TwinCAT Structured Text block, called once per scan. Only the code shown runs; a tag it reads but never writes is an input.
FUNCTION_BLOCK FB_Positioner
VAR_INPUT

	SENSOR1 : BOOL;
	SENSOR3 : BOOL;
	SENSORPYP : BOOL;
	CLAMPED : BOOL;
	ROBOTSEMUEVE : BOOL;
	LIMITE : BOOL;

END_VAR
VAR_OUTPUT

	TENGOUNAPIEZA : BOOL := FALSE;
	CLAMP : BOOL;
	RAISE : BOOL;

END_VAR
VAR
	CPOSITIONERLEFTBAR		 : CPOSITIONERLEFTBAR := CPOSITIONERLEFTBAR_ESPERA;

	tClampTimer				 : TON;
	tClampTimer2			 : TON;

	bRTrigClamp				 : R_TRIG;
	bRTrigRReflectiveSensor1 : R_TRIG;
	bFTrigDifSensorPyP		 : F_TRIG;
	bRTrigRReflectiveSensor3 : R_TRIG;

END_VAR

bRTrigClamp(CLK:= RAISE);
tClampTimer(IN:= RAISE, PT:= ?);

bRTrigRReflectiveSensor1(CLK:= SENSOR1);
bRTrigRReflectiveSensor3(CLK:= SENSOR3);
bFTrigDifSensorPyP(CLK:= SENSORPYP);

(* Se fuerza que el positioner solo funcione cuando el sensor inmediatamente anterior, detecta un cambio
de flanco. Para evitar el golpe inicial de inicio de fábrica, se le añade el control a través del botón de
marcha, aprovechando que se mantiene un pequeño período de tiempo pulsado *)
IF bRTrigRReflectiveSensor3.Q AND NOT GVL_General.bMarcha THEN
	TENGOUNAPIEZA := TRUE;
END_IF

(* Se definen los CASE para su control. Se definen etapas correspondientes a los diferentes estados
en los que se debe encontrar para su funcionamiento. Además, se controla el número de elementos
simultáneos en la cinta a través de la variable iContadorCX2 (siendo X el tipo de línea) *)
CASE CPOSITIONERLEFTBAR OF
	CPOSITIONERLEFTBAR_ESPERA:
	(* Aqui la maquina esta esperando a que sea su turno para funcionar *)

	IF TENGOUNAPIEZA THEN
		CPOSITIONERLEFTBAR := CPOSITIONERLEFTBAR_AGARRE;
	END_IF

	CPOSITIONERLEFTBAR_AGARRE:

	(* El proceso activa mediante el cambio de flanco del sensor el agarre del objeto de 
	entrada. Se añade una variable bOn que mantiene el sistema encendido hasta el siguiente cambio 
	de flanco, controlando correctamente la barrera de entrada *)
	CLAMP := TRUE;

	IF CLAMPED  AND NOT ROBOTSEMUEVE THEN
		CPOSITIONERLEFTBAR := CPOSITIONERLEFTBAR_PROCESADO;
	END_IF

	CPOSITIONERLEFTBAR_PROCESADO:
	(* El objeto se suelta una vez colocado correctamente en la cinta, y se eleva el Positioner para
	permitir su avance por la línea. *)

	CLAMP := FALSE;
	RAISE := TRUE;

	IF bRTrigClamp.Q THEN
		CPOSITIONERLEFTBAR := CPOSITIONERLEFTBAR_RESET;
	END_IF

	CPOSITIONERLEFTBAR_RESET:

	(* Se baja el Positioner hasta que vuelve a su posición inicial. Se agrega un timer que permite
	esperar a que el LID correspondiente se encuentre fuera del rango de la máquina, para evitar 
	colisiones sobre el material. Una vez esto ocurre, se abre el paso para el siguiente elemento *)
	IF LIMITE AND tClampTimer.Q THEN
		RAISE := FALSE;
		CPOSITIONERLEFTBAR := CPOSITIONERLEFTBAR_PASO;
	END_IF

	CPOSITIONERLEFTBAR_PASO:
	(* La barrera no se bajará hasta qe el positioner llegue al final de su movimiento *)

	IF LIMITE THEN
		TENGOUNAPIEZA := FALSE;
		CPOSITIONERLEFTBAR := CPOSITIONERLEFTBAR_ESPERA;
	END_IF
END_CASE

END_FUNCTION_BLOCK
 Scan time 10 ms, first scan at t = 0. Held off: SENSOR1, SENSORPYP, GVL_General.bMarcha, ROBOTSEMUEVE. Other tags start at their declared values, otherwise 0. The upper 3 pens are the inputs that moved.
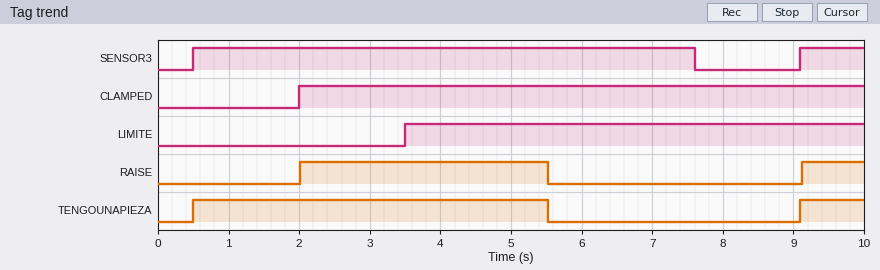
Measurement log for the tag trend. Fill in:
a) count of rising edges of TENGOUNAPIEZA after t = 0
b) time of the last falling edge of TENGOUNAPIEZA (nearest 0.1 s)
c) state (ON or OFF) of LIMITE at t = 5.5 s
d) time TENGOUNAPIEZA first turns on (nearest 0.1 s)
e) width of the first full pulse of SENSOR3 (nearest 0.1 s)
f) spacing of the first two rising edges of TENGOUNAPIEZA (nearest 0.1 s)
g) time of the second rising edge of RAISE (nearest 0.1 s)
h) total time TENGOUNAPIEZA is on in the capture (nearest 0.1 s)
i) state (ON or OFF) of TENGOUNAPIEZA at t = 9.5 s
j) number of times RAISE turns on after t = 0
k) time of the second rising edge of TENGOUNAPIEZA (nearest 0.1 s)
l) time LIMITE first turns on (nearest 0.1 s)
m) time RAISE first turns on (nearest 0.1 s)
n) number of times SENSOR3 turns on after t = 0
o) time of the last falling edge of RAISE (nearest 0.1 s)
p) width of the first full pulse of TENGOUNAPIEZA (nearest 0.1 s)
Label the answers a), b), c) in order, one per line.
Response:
a) 2
b) 5.5 s
c) ON
d) 0.5 s
e) 7.1 s
f) 8.6 s
g) 9.1 s
h) 5.9 s
i) ON
j) 2
k) 9.1 s
l) 3.5 s
m) 2.0 s
n) 2
o) 5.5 s
p) 5.0 s
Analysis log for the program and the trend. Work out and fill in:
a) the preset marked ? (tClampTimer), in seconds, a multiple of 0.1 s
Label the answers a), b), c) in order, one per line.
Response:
a) 3.5 s
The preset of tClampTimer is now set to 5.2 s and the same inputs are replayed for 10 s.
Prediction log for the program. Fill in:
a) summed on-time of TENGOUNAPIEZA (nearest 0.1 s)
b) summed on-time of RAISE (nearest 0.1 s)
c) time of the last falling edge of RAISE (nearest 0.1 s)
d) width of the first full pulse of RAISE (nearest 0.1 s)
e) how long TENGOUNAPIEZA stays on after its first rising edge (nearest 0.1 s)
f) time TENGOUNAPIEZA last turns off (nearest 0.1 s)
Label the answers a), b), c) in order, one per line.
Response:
a) 7.6 s
b) 6.1 s
c) 7.2 s
d) 5.2 s
e) 6.7 s
f) 7.2 s
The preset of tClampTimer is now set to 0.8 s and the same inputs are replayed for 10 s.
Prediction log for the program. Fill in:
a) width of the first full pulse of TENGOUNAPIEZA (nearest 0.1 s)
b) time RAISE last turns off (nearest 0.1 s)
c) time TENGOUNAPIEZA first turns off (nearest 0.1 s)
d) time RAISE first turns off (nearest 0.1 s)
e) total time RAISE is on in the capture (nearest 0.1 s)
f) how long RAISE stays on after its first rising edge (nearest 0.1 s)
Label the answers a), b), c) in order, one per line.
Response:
a) 3.0 s
b) 9.9 s
c) 3.5 s
d) 3.5 s
e) 2.3 s
f) 1.5 s
